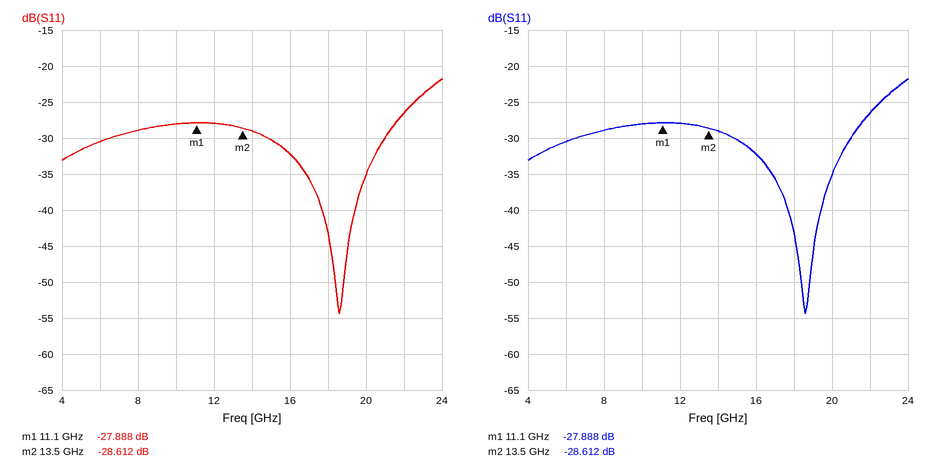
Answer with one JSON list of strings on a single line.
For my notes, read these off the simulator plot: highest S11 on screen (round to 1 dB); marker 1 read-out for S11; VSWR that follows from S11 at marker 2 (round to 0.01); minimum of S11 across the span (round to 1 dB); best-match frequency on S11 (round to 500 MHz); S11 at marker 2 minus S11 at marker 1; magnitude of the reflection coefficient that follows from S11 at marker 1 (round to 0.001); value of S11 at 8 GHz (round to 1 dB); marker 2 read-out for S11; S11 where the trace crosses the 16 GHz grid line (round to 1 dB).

["-22 dB", "-27.888 dB", "1.08", "-54 dB", "18.5 GHz", "-0.724 dB", "0.040", "-29 dB", "-28.612 dB", "-32 dB"]
